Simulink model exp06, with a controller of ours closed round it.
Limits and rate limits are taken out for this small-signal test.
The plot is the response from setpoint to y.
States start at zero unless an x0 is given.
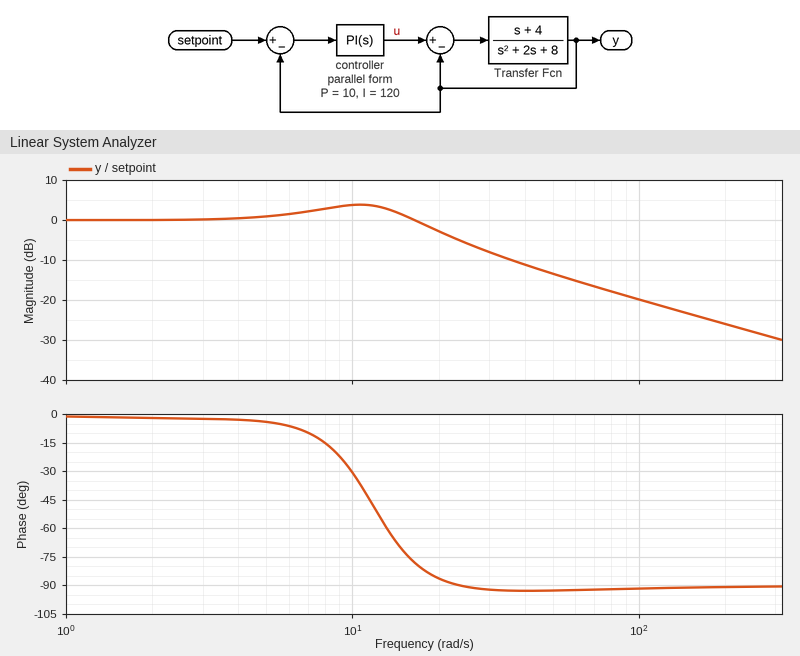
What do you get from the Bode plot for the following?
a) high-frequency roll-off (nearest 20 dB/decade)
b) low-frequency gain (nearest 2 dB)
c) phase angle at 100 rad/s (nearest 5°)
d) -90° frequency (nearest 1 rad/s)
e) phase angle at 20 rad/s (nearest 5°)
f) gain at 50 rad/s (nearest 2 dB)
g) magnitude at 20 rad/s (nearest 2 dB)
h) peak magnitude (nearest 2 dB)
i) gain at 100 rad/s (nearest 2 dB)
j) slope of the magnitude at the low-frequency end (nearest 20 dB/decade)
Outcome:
-20 dB/decade
0 dB
-90°
24 rad/s
-85°
-14 dB
-2 dB
4 dB
-20 dB
0 dB/decade
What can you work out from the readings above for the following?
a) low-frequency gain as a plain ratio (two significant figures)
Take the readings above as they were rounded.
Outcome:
1.0
